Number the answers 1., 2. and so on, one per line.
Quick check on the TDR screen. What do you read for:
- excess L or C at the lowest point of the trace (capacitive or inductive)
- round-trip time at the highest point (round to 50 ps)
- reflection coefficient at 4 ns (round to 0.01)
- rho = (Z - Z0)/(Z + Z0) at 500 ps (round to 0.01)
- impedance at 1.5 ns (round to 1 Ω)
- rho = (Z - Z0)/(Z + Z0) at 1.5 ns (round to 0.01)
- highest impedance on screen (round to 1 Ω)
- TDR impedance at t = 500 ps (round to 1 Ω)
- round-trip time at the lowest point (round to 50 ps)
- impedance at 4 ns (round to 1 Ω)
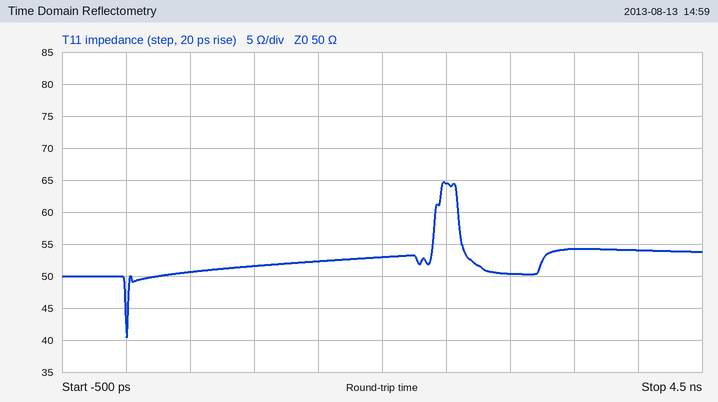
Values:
1. capacitive
2. 2.50 ns
3. +0.04
4. +0.01
5. 52 Ω
6. +0.02
7. 65 Ω
8. 51 Ω
9. 0 ps
10. 54 Ω
